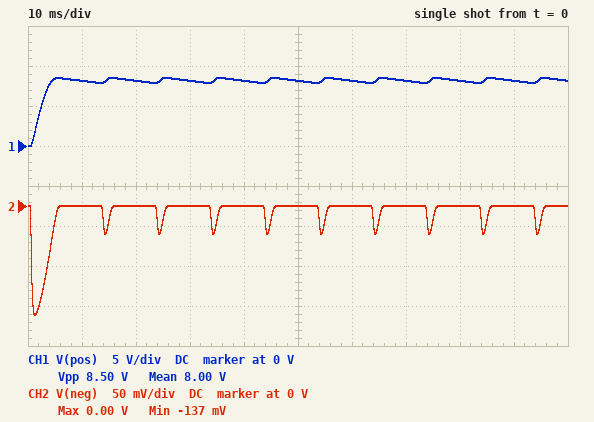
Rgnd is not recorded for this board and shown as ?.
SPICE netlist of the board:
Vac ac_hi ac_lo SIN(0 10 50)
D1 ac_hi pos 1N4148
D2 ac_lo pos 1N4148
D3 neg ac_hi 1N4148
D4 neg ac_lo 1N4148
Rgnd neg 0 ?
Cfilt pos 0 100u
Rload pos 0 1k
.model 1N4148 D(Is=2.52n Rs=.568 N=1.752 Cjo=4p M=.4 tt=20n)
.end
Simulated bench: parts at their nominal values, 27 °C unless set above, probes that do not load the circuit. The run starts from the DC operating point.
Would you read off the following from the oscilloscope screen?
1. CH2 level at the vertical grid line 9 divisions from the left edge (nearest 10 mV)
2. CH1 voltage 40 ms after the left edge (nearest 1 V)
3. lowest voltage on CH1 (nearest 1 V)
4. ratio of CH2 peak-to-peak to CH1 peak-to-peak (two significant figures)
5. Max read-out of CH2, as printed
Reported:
0 V
8 V
0 V
0.016
0.00 V
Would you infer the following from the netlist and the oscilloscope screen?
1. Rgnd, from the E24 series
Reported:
0.47 Ω
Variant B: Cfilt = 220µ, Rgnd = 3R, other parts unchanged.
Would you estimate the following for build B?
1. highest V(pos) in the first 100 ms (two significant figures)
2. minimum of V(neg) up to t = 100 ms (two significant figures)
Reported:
8.3 V
-1.5 V
